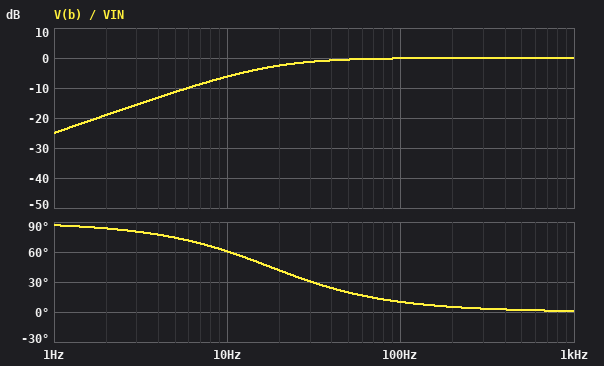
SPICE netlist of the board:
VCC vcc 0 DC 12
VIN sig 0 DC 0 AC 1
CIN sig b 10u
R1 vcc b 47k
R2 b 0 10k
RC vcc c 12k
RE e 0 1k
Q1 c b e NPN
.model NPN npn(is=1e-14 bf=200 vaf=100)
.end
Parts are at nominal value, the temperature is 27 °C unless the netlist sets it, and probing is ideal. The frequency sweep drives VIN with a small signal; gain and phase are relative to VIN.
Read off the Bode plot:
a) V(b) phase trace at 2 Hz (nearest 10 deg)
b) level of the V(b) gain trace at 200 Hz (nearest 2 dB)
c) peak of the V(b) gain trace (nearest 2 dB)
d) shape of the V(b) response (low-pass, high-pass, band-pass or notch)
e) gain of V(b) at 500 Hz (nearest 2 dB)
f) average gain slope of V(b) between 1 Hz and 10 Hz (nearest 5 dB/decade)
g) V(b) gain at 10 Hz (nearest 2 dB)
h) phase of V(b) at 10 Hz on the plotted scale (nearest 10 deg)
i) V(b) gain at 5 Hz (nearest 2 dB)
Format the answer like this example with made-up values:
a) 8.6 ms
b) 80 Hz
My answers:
a) 80 deg
b) 0 dB
c) 0 dB
d) high-pass
e) 0 dB
f) 20 dB/decade
g) -6 dB
h) 60 deg
i) -12 dB
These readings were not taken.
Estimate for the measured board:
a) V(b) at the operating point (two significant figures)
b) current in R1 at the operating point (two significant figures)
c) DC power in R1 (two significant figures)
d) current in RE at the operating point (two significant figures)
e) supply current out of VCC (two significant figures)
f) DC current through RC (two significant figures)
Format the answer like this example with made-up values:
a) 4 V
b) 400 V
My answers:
a) 1.6 V
b) 220 µA
c) 2.3 mW
d) 970 µA
e) 1.1 mA
f) 910 µA
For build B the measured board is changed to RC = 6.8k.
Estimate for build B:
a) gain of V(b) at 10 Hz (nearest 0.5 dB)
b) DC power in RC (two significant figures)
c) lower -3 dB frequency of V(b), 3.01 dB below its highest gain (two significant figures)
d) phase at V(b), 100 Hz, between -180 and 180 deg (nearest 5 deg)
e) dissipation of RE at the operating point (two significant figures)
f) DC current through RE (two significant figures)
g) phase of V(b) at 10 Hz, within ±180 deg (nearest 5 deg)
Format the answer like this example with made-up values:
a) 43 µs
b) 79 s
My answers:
a) 0 dB
b) 13 mW
c) 2.0 Hz
d) 0 deg
e) 1.9 mW
f) 1.4 mA
g) 10 deg
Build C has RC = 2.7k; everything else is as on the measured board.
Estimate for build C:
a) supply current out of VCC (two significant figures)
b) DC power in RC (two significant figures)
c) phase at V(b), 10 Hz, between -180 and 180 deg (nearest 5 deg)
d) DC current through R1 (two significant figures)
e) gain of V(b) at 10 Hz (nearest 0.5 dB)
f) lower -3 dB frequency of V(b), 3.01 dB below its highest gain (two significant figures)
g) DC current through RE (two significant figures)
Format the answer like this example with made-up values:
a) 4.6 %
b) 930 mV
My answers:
a) 1.6 mA
b) 5.2 mW
c) 10 deg
d) 210 µA
e) 0 dB
f) 2.0 Hz
g) 1.4 mA
